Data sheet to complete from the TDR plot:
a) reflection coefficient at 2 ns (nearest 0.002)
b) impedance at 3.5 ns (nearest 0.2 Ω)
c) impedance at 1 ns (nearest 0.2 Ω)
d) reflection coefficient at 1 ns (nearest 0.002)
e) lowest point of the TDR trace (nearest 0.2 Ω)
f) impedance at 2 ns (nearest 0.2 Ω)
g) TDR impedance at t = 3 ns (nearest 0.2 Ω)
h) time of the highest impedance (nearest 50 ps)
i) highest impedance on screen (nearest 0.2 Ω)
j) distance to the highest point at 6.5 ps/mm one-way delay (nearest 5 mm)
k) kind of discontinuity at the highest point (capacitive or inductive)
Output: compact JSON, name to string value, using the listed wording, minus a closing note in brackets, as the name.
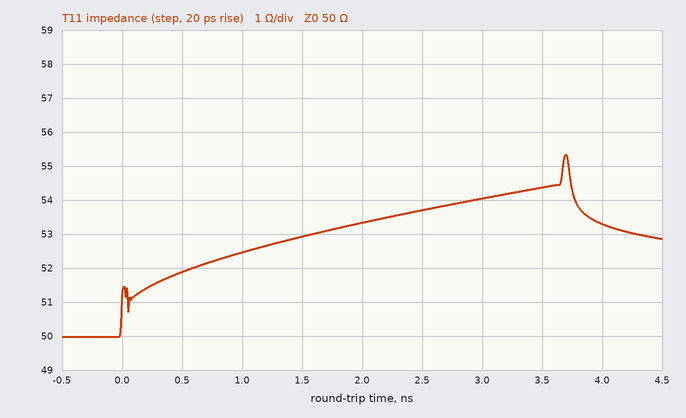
{"reflection coefficient at 2 ns": "+0.032", "impedance at 3.5 ns": "54.4 Ω", "impedance at 1 ns": "52.4 Ω", "reflection coefficient at 1 ns": "+0.024", "lowest point of the TDR trace": "50.0 Ω", "impedance at 2 ns": "53.4 Ω", "TDR impedance at t = 3 ns": "54.0 Ω", "time of the highest impedance": "3.70 ns", "highest impedance on screen": "55.4 Ω", "distance to the highest point at 6.5 ps/mm one-way delay": "285 mm", "kind of discontinuity at the highest point": "inductive"}
